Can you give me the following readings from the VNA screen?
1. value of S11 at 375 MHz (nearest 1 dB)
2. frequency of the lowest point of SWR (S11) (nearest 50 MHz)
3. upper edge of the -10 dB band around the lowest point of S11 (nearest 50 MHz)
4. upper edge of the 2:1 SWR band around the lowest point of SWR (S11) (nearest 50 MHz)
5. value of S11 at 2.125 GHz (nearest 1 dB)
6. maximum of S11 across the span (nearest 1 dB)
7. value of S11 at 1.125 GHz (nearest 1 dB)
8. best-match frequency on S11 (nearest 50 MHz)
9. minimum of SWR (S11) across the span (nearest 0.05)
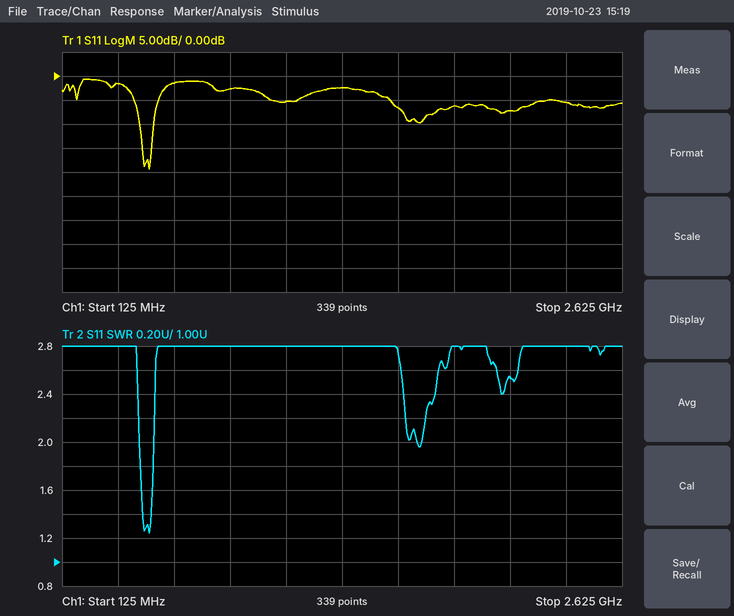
-2 dB
500 MHz
550 MHz
550 MHz
-7 dB
-1 dB
-5 dB
500 MHz
1.25
